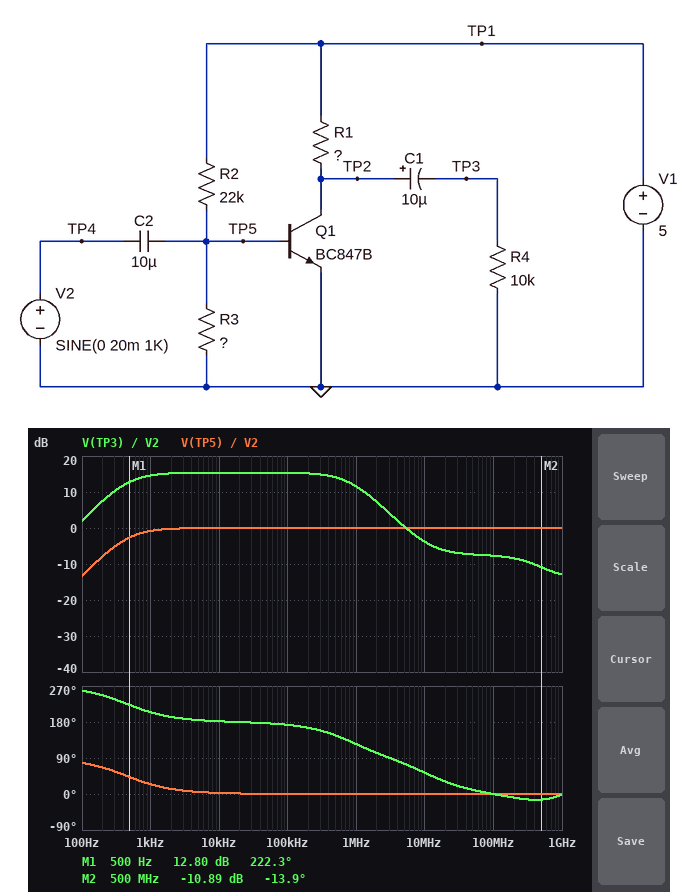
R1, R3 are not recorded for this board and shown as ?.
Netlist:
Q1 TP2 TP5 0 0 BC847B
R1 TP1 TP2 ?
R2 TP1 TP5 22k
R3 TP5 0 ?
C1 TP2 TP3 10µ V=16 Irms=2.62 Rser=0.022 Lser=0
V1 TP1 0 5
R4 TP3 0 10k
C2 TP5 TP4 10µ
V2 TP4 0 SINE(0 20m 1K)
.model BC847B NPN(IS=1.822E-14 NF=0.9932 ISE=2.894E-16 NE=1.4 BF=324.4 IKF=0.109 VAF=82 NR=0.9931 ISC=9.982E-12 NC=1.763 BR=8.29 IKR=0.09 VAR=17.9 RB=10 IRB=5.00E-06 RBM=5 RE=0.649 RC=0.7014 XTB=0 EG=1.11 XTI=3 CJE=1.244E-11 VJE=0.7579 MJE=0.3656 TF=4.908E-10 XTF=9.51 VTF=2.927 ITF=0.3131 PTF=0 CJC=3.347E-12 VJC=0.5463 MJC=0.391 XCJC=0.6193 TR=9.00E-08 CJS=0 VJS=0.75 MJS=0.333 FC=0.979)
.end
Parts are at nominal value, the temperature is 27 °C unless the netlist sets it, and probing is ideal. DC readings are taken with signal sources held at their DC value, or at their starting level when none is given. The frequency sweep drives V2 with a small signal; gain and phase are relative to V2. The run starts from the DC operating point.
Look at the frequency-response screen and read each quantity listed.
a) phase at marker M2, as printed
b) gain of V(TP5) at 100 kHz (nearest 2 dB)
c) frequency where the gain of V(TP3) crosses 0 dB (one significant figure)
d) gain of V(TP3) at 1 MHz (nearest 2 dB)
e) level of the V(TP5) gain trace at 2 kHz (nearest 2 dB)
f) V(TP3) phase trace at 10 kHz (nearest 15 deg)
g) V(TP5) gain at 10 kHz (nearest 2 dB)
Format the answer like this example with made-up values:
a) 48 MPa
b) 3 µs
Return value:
a) -13.9 deg
b) 0 dB
c) 5 MHz
d) 12 dB
e) 0 dB
f) 180 deg
g) 0 dB
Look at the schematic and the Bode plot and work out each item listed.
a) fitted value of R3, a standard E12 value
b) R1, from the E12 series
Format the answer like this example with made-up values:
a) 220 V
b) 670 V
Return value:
a) 12 kΩ
b) 680 Ω
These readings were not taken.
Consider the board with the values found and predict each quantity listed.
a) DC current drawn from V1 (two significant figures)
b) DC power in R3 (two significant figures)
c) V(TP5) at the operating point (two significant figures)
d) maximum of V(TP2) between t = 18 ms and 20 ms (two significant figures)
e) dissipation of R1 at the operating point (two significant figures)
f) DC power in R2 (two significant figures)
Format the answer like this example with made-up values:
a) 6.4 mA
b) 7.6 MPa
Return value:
a) 7.4 mA
b) 41 µW
c) 700 mV
d) 2.6 V
e) 36 mW
f) 840 µW
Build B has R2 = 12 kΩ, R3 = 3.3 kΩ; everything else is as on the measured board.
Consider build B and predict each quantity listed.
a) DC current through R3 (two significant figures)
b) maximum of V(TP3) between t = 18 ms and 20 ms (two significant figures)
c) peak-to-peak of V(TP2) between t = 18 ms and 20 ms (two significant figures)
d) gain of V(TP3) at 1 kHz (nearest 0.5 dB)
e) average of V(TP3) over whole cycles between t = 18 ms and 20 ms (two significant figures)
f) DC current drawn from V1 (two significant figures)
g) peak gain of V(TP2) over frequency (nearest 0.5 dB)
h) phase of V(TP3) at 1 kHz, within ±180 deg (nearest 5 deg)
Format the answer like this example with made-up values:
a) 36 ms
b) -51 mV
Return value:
a) 210 µA
b) 2.3 V
c) 2.5 V
d) 14.0 dB
e) 780 mV
f) 7.6 mA
g) 14.5 dB
h) -155 deg
